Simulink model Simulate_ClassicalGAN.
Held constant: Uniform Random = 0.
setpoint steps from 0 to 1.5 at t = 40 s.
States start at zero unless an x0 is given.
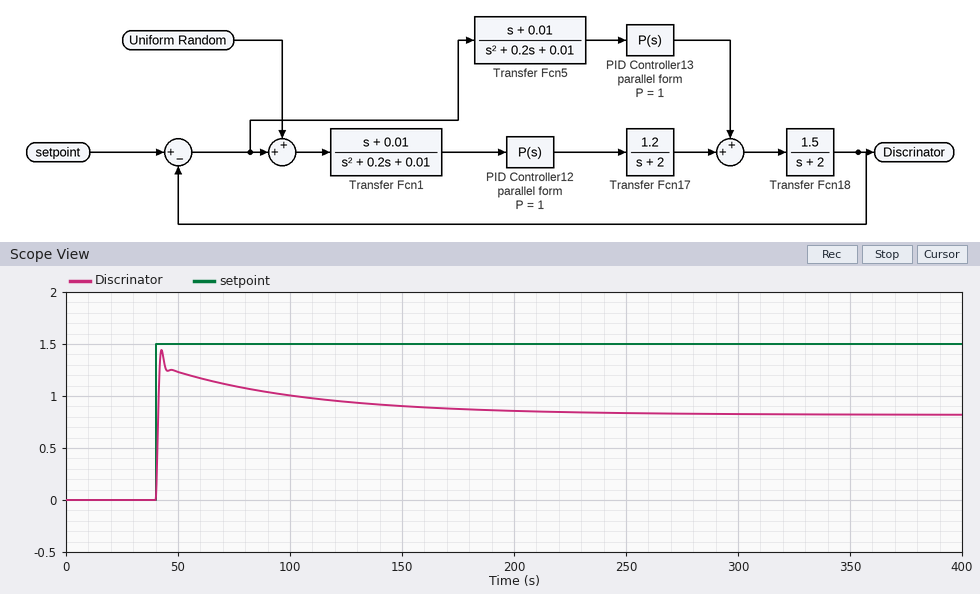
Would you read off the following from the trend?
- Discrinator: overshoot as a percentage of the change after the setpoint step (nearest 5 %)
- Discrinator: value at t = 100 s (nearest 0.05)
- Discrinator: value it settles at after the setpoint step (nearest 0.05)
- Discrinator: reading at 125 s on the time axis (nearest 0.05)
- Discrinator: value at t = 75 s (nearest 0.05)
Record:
75 %
1.00
0.80
0.95
1.10
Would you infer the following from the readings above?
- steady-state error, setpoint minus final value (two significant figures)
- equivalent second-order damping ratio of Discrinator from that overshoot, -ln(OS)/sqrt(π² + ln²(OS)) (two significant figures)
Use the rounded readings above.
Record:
0.70
0.091
